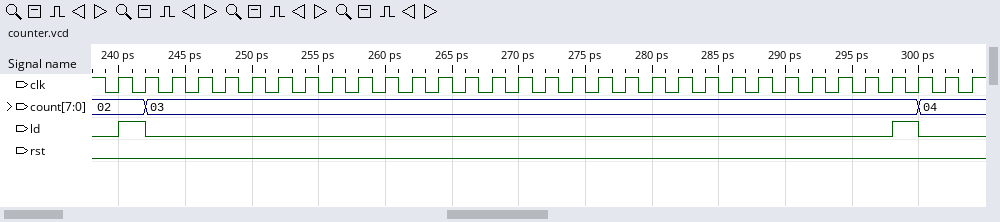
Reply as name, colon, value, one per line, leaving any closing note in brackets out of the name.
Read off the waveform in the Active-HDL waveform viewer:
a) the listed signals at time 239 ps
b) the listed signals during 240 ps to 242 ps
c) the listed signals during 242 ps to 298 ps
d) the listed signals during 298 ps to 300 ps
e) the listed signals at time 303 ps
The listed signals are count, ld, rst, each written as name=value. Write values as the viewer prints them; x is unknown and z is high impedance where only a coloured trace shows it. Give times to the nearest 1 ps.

the listed signals at time 239 ps: count=02, ld=0, rst=0
the listed signals during 240 ps to 242 ps: count=02, ld=1, rst=0
the listed signals during 242 ps to 298 ps: count=03, ld=0, rst=0
the listed signals during 298 ps to 300 ps: count=03, ld=1, rst=0
the listed signals at time 303 ps: count=04, ld=0, rst=0
